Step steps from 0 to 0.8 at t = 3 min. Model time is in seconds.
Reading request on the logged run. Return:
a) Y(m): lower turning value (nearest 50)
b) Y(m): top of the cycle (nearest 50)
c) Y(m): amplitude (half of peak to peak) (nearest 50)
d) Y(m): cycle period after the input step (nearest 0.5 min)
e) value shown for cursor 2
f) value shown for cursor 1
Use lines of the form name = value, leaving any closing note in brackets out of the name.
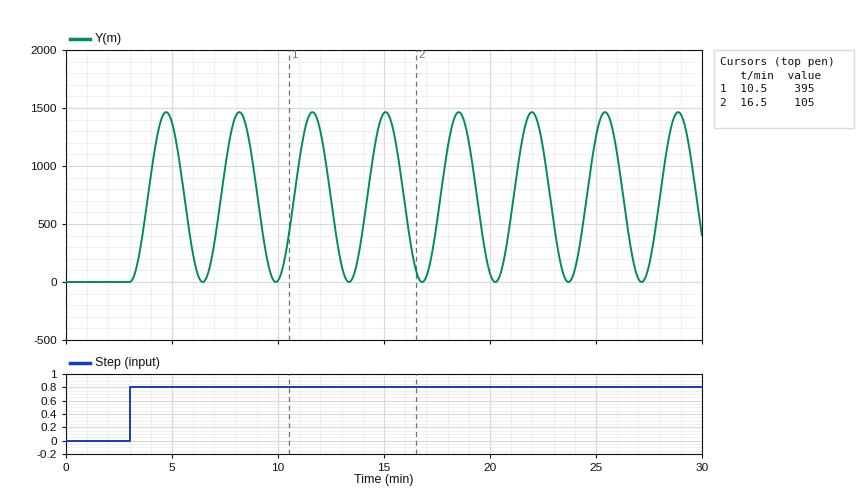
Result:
Y(m): lower turning value = 0
Y(m): top of the cycle = 1450
Y(m): amplitude (half of peak to peak) = 750
Y(m): cycle period after the input step = 3.5 min
value shown for cursor 2 = 105
value shown for cursor 1 = 395
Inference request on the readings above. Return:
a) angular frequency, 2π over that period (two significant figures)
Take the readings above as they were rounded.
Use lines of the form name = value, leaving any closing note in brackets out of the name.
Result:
angular frequency, 2π over that period = 1.8 rad/min
